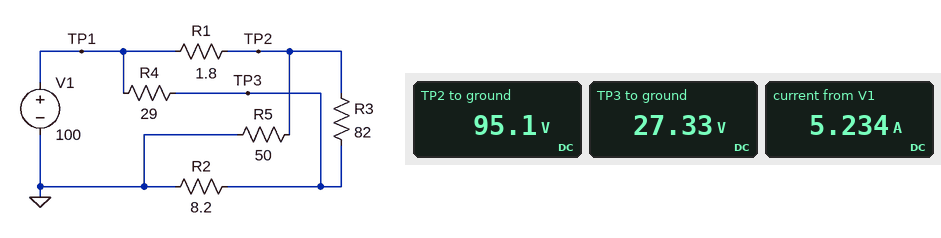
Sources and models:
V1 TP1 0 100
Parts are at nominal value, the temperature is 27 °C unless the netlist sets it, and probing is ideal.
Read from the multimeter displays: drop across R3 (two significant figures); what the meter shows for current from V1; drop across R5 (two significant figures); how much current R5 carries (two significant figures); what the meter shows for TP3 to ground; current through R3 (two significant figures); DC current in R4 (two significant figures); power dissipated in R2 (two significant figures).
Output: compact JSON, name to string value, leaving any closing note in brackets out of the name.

{"drop across R3": "68 V", "what the meter shows for current from V1": "5.234 A", "drop across R5": "95 V", "how much current R5 carries": "1.9 A", "what the meter shows for TP3 to ground": "27.33 V", "current through R3": "830 mA", "DC current in R4": "2.5 A", "power dissipated in R2": "91 W"}
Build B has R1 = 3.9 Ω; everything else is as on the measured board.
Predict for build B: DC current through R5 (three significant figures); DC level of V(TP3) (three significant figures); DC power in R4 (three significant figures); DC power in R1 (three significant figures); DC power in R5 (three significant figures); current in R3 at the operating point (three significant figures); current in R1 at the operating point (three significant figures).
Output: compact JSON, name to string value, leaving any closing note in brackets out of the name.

{"DC current through R5": "1.80 A", "DC level of V(TP3)": "27.0 V", "DC power in R4": "184 W", "DC power in R1": "25.7 W", "DC power in R5": "162 W", "current in R3 at the operating point": "769 mA", "current in R1 at the operating point": "2.57 A"}
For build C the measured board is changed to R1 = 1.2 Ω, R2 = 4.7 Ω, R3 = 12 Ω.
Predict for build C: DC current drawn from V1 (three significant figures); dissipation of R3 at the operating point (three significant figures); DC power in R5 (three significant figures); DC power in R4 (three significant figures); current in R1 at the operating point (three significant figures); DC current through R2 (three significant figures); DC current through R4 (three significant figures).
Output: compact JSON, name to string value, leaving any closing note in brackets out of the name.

{"DC current drawn from V1": "8.99 A", "dissipation of R3 at the operating point": "284 W", "DC power in R5": "169 W", "DC power in R4": "152 W", "current in R1 at the operating point": "6.70 A", "DC current through R2": "7.15 A", "DC current through R4": "2.29 A"}
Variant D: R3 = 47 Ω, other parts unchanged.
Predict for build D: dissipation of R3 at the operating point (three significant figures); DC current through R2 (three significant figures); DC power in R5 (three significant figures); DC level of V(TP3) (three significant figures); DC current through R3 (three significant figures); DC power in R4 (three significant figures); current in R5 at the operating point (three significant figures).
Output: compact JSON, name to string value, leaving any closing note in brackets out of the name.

{"dissipation of R3 at the operating point": "85.8 W", "DC current through R2": "3.74 A", "DC power in R5": "177 W", "DC level of V(TP3)": "30.7 V", "DC current through R3": "1.35 A", "DC power in R4": "166 W", "current in R5 at the operating point": "1.88 A"}
